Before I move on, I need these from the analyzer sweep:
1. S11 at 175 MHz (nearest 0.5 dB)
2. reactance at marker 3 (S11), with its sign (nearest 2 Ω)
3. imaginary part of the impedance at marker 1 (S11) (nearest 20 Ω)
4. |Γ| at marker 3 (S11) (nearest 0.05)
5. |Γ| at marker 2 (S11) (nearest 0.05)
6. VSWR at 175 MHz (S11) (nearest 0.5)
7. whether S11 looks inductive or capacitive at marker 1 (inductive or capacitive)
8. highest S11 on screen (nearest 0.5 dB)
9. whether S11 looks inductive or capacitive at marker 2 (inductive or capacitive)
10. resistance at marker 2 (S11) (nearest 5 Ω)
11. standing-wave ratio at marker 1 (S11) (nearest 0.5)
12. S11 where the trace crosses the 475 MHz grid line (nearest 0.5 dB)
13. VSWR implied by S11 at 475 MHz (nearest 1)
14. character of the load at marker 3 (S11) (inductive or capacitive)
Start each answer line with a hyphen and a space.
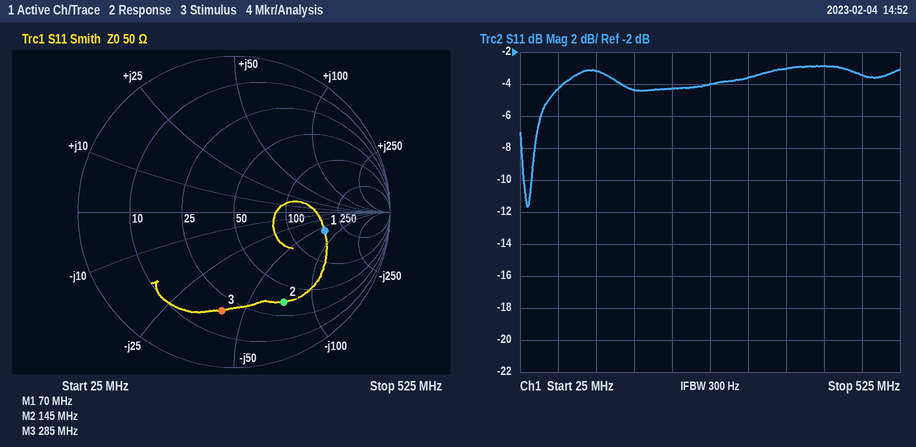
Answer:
- -4.5 dB
- -40 Ω
- -60 Ω
- 0.65
- 0.65
- 4.0
- capacitive
- -3.0 dB
- capacitive
- 35 Ω
- 4.0
- -3.5 dB
- 5
- capacitive
